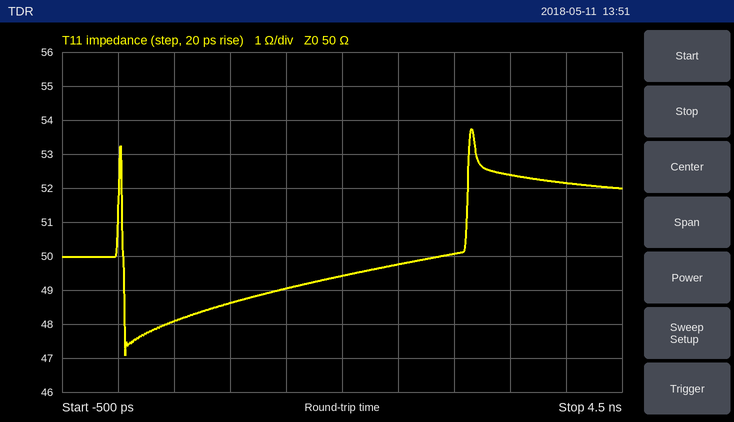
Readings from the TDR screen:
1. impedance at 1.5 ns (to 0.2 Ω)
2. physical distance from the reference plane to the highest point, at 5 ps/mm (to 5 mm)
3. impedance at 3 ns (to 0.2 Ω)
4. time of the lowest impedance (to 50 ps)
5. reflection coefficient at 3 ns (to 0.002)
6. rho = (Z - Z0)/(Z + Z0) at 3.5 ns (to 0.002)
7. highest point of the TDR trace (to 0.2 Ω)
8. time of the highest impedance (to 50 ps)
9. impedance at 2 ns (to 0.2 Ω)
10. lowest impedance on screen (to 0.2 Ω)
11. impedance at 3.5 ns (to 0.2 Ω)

49.0 Ω
315 mm
50.0 Ω
50 ps
0.000
+0.024
53.8 Ω
3.15 ns
49.4 Ω
47.0 Ω
52.4 Ω
